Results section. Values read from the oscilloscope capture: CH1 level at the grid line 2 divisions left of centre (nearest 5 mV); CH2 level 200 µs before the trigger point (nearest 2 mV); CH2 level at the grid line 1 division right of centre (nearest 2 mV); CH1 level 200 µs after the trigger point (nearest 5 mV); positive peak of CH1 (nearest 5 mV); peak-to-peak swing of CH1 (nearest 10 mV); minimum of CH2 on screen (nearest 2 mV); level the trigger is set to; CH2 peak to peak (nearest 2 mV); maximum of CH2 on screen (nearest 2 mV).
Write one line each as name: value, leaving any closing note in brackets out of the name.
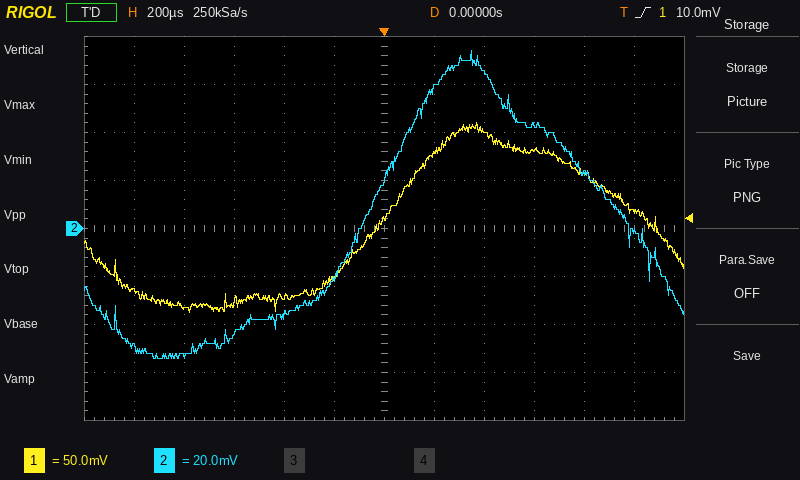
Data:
CH1 level at the grid line 2 divisions left of centre: -70 mV
CH2 level 200 µs before the trigger point: -20 mV
CH2 level at the grid line 1 division right of centre: 58 mV
CH1 level 200 µs after the trigger point: 80 mV
positive peak of CH1: 110 mV
peak-to-peak swing of CH1: 200 mV
minimum of CH2 on screen: -54 mV
level the trigger is set to: 10.0 mV
CH2 peak to peak: 128 mV
maximum of CH2 on screen: 74 mV
